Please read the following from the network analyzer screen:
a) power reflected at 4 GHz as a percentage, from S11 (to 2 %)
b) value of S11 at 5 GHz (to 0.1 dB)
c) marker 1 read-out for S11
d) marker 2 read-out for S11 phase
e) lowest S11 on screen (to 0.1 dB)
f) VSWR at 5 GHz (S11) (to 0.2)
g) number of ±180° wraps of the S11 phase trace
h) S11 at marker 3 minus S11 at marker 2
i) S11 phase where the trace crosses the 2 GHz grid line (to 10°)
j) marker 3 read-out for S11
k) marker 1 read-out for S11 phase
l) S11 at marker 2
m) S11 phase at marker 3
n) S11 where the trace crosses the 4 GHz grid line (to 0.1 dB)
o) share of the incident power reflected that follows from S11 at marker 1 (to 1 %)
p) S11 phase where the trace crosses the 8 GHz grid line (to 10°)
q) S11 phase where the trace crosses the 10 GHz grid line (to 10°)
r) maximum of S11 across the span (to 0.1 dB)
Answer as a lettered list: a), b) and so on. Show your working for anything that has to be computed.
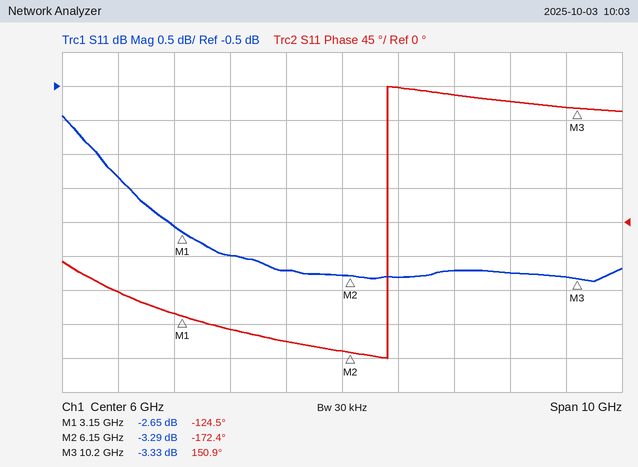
a) 10^(-3/10) ≈ 50 %
b) -3.2 dB
c) -2.65 dB
d) -172.4°
e) -3.4 dB
f) |Γ| = 10^(-3.2/20) = 0.6918; VSWR = (1 + 0.6918)/(1 − 0.6918) ≈ 5.49, so 5.4 to the nearest 0.2
g) 1
h) -3.33 − (-3.29) = -0.04 dB
i) -90°
j) -3.33 dB
k) -124.5°
l) -3.29 dB
m) 150.9°
n) -3.0 dB
o) 10^(-2.65/10) ≈ 54 %
p) 170°
q) 150°
r) -0.9 dB
